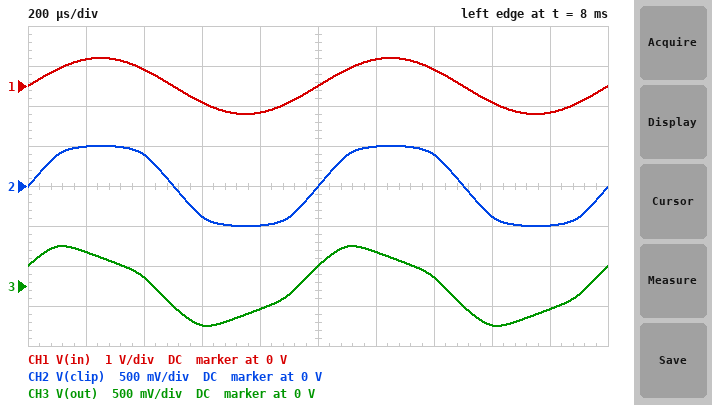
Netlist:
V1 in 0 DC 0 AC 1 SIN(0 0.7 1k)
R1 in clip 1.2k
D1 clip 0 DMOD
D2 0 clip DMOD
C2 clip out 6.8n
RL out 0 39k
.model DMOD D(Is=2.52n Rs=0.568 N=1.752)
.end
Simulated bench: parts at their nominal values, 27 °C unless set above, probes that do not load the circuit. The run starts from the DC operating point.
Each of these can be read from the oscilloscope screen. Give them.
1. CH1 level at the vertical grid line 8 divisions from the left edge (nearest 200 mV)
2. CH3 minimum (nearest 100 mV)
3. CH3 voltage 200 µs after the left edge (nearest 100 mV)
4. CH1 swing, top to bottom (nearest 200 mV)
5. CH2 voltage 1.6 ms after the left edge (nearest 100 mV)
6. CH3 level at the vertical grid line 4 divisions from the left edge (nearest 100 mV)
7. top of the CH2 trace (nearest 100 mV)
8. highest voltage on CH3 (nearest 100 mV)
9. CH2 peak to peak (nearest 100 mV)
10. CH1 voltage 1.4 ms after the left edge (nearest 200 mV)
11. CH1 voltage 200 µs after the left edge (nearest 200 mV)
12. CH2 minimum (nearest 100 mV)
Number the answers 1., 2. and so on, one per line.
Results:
1. -400 mV
2. -500 mV
3. 400 mV
4. 1.4 V
5. -400 mV
6. -300 mV
7. 500 mV
8. 500 mV
9. 1.0 V
10. 400 mV
11. 600 mV
12. -500 mV
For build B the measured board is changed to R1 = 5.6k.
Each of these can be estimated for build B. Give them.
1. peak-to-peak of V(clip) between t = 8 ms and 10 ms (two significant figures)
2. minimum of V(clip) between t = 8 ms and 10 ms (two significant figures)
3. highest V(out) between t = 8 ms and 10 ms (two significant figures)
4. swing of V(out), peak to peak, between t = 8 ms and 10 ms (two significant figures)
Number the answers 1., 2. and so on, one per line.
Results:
1. 870 mV
2. -440 mV
3. 440 mV
4. 880 mV
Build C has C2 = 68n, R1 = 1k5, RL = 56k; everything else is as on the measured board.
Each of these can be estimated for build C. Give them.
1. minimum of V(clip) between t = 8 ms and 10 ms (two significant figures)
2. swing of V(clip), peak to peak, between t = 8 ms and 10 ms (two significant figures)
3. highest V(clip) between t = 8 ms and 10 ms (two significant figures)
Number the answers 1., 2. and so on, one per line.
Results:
1. -490 mV
2. 980 mV
3. 490 mV
